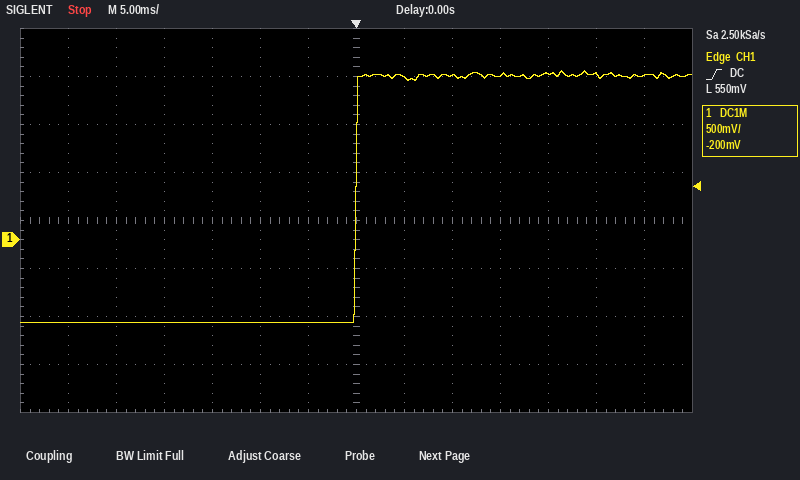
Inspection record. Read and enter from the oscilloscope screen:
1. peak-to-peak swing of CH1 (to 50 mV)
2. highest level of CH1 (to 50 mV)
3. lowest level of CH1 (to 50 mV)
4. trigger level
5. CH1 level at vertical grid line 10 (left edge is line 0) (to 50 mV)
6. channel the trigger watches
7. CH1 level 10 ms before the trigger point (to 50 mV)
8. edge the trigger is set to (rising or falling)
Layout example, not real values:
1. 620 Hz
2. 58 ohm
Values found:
1. 2.60 V
2. 1.75 V
3. -850 mV
4. 550 mV
5. 1.70 V
6. CH1
7. -850 mV
8. rising
